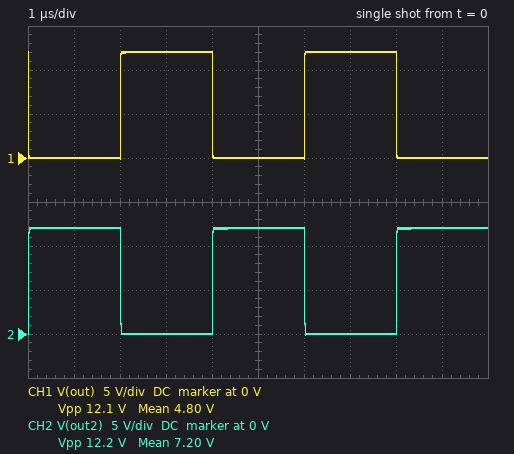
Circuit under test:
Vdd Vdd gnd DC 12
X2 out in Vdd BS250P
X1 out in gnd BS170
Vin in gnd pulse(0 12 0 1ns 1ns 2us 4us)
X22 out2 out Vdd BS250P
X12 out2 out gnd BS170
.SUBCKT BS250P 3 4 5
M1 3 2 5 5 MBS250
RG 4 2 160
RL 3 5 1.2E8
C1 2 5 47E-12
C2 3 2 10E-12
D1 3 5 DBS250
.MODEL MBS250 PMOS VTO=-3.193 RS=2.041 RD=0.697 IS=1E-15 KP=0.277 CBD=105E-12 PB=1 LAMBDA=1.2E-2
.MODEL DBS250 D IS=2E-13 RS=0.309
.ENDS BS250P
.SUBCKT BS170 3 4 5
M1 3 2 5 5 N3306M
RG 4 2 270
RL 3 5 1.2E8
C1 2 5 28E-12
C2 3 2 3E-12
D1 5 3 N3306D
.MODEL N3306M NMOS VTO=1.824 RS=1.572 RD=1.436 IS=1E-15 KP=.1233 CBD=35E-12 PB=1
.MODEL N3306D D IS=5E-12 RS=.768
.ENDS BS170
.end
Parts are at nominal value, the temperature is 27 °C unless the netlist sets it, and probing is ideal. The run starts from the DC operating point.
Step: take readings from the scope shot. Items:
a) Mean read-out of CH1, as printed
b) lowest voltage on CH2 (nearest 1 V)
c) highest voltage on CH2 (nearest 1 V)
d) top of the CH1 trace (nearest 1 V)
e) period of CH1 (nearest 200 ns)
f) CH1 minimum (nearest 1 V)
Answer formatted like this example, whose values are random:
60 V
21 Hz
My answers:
4.80 V
0 V
12 V
12 V
4.0 µs
0 V
